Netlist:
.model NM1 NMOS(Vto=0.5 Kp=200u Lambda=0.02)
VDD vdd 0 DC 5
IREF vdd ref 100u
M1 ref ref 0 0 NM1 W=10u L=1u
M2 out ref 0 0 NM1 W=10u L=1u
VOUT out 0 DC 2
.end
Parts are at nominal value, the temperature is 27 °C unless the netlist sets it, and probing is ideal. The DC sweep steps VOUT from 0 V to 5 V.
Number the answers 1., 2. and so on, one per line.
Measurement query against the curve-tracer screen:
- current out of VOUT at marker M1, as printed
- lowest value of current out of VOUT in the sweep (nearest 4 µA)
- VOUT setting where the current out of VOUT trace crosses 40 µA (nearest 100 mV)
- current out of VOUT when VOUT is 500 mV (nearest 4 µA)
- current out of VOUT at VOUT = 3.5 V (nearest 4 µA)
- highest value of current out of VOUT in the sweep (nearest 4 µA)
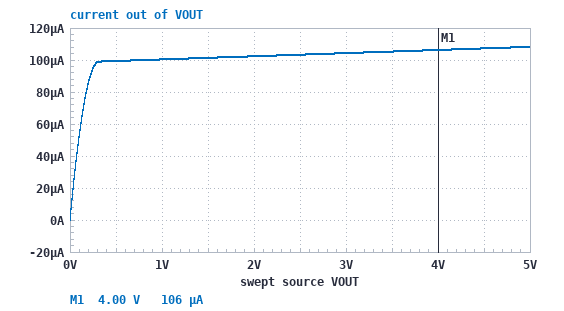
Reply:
1. 106 µA
2. 0 A
3. 100 mV
4. 100 µA
5. 104 µA
6. 108 µA
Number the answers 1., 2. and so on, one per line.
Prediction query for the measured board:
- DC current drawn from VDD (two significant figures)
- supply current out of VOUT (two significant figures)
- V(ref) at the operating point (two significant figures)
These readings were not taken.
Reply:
1. 100 µA
2. 100 µA
3. 810 mV
